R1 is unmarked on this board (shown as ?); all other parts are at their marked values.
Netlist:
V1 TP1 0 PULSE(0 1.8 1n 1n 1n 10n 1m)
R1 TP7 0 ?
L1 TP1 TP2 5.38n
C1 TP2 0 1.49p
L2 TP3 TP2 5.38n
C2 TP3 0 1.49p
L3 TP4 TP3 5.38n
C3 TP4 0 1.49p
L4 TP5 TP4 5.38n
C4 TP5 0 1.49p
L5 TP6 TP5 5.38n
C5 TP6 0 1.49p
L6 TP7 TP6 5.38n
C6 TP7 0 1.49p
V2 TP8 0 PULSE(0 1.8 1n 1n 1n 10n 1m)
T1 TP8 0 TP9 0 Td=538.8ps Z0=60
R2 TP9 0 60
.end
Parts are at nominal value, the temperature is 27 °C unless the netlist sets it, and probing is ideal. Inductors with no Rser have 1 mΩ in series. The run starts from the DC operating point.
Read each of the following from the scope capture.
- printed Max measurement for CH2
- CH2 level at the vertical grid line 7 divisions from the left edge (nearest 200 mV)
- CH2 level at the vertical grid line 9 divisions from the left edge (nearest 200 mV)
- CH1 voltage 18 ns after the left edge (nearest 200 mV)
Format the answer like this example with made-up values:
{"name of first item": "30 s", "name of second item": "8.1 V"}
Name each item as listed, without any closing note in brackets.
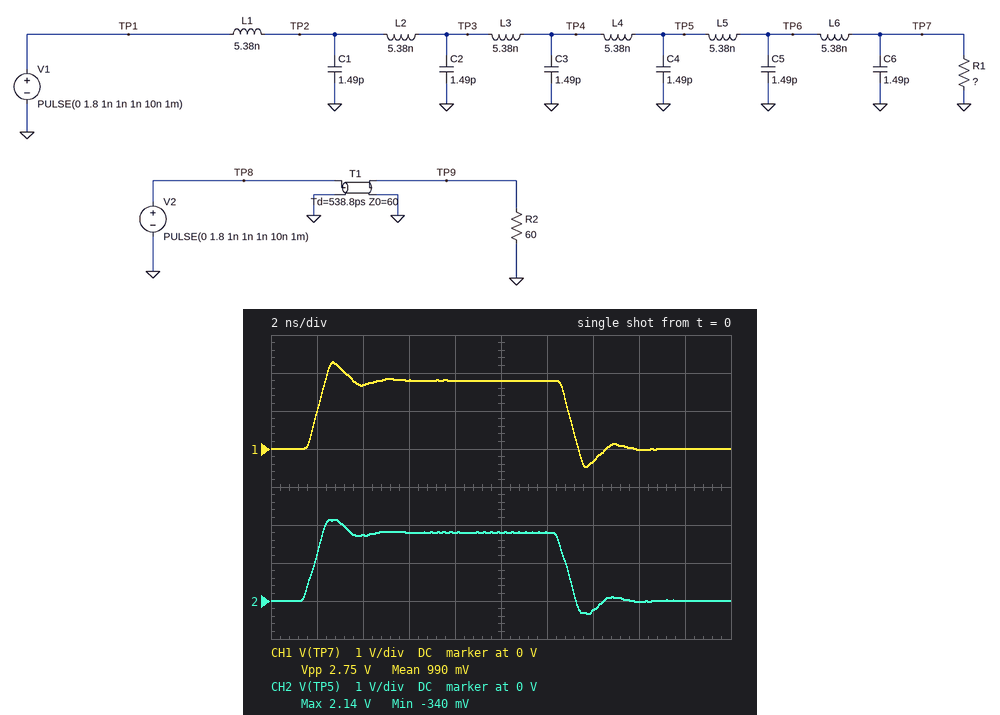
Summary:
{"printed Max measurement for CH2": "2.14 V", "CH2 level at the vertical grid line 7 divisions from the left edge": "-200 mV", "CH2 level at the vertical grid line 9 divisions from the left edge": "0 V", "CH1 voltage 18 ns after the left edge": "0 V"}
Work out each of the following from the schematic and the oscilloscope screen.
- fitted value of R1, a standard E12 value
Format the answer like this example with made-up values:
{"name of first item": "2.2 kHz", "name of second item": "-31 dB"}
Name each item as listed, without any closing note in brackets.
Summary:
{"fitted value of R1, a standard E12 value": "100 Ω"}
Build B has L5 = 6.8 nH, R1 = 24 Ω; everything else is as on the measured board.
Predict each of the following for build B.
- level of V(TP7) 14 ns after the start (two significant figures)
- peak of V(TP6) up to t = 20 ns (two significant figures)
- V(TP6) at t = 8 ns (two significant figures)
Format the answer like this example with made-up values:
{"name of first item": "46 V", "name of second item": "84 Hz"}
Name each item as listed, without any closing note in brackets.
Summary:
{"level of V(TP7) 14 ns after the start": "630 mV", "peak of V(TP6) up to t = 20 ns": "1.8 V", "V(TP6) at t = 8 ns": "1.8 V"}
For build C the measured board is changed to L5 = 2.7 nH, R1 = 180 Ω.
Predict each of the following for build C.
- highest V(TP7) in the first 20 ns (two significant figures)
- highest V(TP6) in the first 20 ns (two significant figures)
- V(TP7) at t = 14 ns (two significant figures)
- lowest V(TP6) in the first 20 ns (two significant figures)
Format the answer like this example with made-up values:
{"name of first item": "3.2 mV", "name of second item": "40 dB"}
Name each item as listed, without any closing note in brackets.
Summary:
{"highest V(TP7) in the first 20 ns": "2.7 V", "highest V(TP6) in the first 20 ns": "2.6 V", "V(TP7) at t = 14 ns": "-540 mV", "lowest V(TP6) in the first 20 ns": "-800 mV"}
